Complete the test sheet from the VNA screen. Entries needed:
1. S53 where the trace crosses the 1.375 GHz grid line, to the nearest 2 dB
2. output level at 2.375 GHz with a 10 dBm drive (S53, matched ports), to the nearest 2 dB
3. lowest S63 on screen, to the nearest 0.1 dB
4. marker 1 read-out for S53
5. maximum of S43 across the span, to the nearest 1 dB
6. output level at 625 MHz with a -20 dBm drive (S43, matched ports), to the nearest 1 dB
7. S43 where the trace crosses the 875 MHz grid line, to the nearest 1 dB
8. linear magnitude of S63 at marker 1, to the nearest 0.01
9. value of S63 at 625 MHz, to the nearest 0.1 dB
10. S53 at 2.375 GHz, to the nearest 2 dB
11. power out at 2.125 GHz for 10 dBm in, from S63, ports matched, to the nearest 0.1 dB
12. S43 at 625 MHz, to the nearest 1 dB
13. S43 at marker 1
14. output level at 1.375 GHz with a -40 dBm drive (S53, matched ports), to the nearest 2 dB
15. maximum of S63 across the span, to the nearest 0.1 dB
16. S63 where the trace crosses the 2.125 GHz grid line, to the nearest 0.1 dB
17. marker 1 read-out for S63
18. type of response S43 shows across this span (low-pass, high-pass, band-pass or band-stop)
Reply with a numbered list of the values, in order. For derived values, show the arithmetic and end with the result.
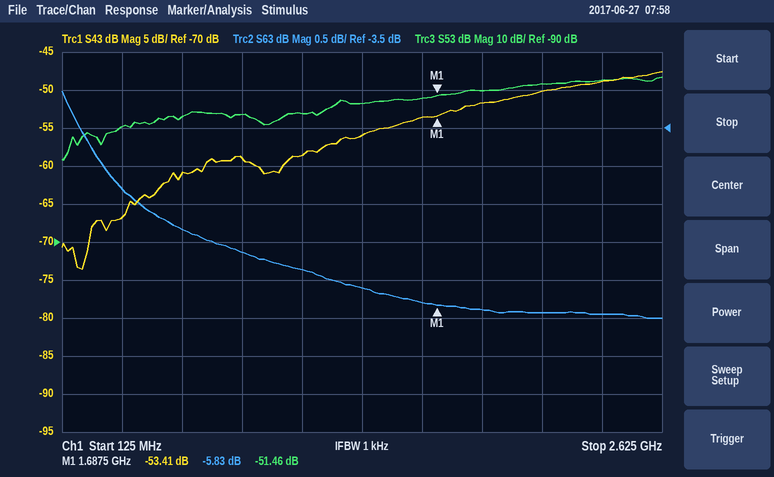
1. -54 dB
2. 10 dBm + (-48 dB) = -38 dBm
3. -6.0 dB
4. -51.46 dB
5. -48 dB
6. -20 dBm + (-61 dB) = -81 dBm
7. -59 dB
8. 10^(-5.83/20) ≈ 0.51
9. -4.8 dB
10. -48 dB
11. 10 dBm + (-5.9 dB) = 4.1 dBm
12. -61 dB
13. -53.41 dB
14. -40 dBm + (-54 dB) = -94 dBm
15. -3.0 dB
16. -5.9 dB
17. -5.83 dB
18. high-pass
